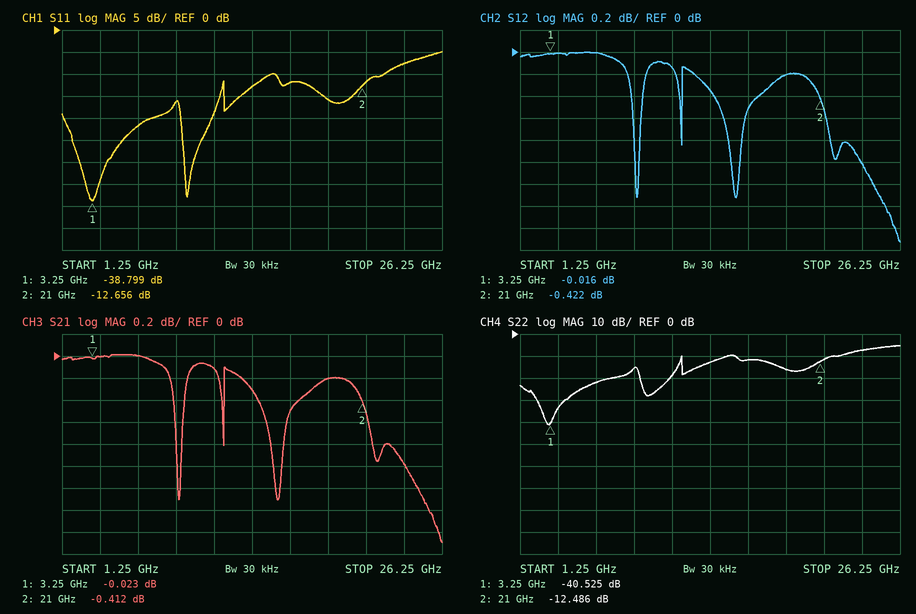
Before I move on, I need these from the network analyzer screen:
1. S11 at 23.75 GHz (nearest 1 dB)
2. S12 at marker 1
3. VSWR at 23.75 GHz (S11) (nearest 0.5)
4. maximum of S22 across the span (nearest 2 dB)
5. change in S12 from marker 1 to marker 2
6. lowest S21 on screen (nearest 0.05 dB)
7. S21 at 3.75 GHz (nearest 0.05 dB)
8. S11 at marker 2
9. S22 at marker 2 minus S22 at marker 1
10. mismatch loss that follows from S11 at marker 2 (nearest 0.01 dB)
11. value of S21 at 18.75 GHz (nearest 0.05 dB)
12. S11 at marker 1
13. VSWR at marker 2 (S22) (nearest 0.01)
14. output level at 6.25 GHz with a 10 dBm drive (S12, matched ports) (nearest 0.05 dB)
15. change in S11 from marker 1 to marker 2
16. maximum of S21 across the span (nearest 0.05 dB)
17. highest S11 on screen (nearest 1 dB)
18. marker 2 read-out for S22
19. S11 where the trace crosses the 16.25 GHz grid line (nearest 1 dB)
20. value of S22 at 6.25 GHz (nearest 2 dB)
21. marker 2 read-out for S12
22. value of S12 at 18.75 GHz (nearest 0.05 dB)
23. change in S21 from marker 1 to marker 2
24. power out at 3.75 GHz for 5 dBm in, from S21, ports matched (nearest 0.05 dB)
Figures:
-8 dB
-0.016 dB
2.5
-6 dB
-0.406 dB
-1.70 dB
0.00 dB
-12.656 dB
28.039 dB
0.24 dB
-0.20 dB
-38.799 dB
1.62
10.00 dBm
26.143 dB
0.00 dB
-5 dB
-12.486 dB
-12 dB
-22 dB
-0.422 dB
-0.20 dB
-0.389 dB
5.00 dBm
